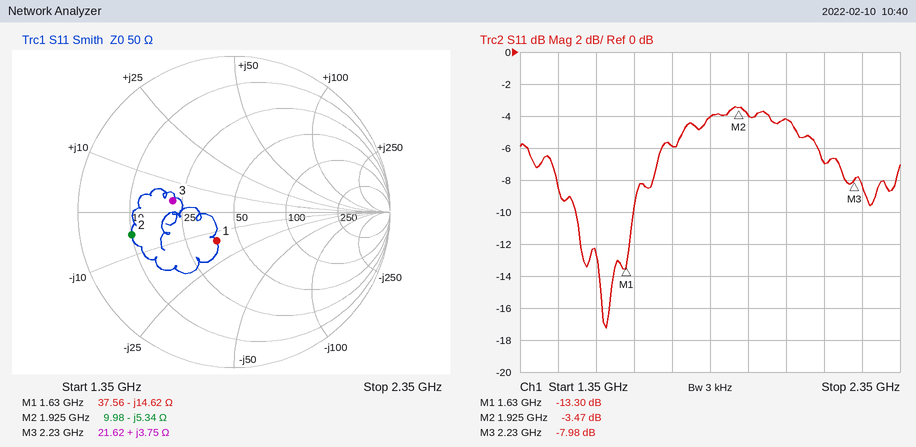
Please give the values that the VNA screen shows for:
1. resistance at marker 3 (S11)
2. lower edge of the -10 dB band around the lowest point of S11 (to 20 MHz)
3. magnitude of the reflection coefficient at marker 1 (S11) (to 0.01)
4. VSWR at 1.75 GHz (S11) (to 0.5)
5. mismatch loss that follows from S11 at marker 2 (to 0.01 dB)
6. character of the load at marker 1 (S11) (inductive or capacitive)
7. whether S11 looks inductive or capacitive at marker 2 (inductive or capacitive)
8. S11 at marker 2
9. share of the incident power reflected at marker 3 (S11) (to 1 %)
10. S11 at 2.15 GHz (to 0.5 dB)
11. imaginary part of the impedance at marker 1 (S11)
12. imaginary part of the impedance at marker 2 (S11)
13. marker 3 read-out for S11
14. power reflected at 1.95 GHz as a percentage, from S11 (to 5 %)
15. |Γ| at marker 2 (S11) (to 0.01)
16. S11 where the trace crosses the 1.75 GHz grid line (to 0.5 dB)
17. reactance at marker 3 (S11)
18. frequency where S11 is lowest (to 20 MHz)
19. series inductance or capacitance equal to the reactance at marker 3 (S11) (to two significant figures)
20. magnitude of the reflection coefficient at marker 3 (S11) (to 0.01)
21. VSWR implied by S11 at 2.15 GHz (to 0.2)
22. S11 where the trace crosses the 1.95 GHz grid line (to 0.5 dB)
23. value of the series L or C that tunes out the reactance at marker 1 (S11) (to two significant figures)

21.62 Ω
1.50 GHz
0.22
3.0
2.59 dB
capacitive
capacitive
-3.47 dB
16 %
-7.0 dB
-14.62 Ω
-5.34 Ω
-7.98 dB
40 %
0.67
-6.0 dB
+3.75 Ω
1.58 GHz
270 pH
0.40
2.6
-4.0 dB
1.4 nH
